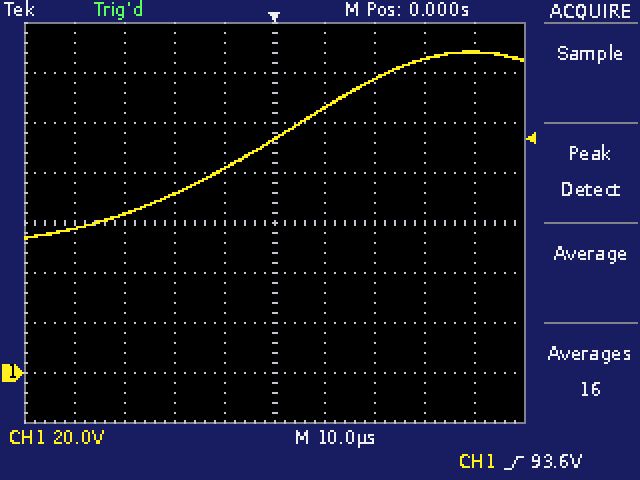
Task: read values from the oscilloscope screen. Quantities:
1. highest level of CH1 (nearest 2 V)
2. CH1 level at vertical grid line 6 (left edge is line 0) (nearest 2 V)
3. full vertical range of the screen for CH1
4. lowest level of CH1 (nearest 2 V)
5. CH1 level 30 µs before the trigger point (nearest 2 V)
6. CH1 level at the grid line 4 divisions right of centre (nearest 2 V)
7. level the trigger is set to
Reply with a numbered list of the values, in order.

1. 128 V
2. 106 V
3. 160 V
4. 54 V
5. 64 V
6. 128 V
7. 93.6 V
